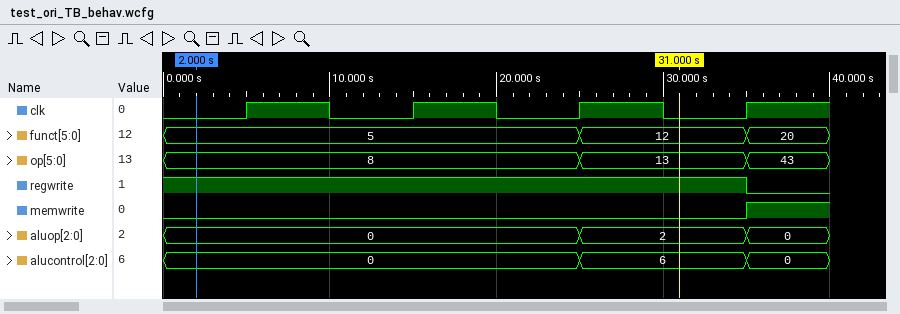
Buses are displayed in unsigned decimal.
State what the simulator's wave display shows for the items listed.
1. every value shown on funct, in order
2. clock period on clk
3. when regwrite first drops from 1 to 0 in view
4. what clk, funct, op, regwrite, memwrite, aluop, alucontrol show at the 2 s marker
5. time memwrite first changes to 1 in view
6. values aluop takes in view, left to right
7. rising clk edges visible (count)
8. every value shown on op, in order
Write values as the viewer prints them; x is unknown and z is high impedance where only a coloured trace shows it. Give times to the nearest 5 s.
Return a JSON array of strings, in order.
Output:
["5, 12, 20", "10 s", "35 s", "clk=0, funct=5, op=8, regwrite=1, memwrite=0, aluop=0, alucontrol=0", "35 s", "0, 2, 0", "4", "8, 13, 43"]
